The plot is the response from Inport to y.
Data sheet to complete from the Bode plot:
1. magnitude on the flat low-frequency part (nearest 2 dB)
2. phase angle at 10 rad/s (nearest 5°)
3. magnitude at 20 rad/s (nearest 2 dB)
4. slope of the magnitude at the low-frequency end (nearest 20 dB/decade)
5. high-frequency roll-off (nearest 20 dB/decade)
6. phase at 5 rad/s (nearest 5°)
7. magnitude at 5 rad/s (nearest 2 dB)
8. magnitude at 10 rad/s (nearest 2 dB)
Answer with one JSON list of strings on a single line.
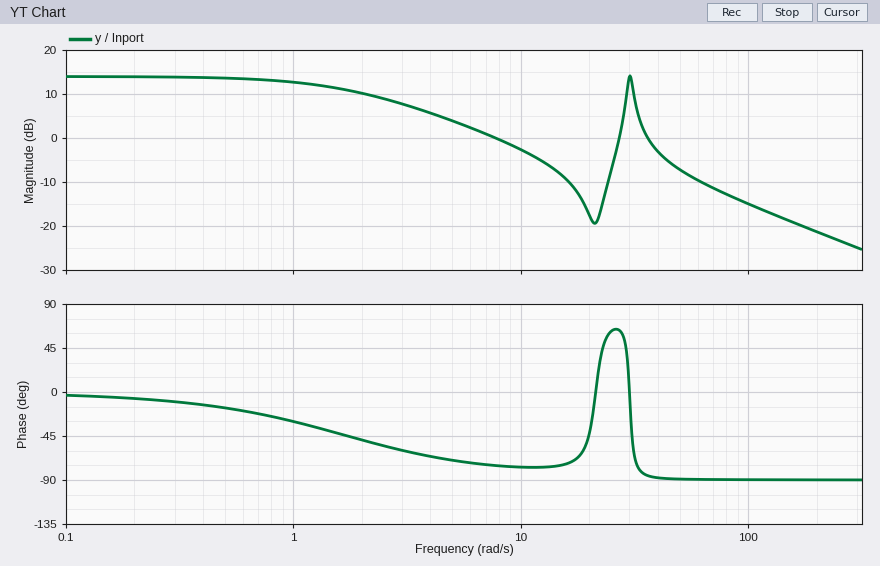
["14 dB", "-75°", "-18 dB", "0 dB/decade", "-20 dB/decade", "-70°", "4 dB", "-2 dB"]
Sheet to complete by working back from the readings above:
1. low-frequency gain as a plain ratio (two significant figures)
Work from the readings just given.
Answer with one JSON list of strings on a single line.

["5.0"]
